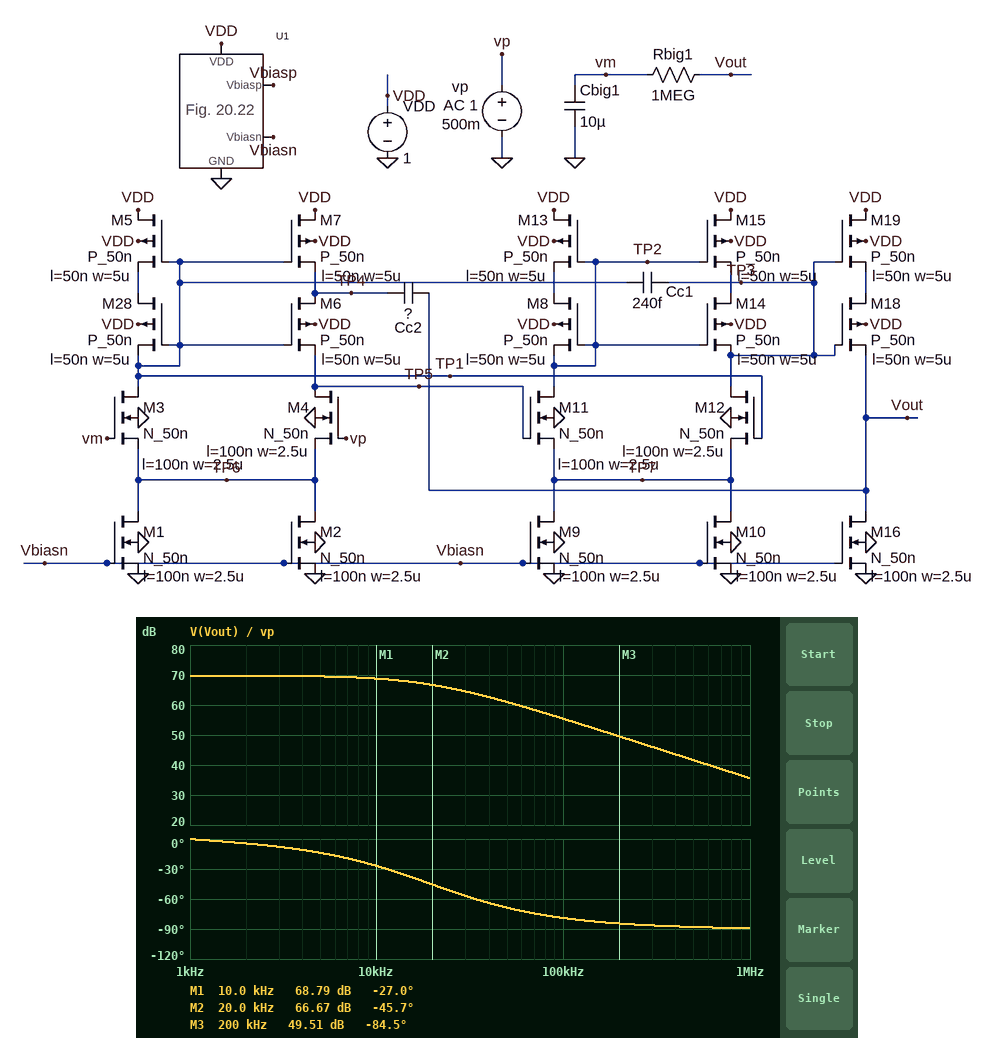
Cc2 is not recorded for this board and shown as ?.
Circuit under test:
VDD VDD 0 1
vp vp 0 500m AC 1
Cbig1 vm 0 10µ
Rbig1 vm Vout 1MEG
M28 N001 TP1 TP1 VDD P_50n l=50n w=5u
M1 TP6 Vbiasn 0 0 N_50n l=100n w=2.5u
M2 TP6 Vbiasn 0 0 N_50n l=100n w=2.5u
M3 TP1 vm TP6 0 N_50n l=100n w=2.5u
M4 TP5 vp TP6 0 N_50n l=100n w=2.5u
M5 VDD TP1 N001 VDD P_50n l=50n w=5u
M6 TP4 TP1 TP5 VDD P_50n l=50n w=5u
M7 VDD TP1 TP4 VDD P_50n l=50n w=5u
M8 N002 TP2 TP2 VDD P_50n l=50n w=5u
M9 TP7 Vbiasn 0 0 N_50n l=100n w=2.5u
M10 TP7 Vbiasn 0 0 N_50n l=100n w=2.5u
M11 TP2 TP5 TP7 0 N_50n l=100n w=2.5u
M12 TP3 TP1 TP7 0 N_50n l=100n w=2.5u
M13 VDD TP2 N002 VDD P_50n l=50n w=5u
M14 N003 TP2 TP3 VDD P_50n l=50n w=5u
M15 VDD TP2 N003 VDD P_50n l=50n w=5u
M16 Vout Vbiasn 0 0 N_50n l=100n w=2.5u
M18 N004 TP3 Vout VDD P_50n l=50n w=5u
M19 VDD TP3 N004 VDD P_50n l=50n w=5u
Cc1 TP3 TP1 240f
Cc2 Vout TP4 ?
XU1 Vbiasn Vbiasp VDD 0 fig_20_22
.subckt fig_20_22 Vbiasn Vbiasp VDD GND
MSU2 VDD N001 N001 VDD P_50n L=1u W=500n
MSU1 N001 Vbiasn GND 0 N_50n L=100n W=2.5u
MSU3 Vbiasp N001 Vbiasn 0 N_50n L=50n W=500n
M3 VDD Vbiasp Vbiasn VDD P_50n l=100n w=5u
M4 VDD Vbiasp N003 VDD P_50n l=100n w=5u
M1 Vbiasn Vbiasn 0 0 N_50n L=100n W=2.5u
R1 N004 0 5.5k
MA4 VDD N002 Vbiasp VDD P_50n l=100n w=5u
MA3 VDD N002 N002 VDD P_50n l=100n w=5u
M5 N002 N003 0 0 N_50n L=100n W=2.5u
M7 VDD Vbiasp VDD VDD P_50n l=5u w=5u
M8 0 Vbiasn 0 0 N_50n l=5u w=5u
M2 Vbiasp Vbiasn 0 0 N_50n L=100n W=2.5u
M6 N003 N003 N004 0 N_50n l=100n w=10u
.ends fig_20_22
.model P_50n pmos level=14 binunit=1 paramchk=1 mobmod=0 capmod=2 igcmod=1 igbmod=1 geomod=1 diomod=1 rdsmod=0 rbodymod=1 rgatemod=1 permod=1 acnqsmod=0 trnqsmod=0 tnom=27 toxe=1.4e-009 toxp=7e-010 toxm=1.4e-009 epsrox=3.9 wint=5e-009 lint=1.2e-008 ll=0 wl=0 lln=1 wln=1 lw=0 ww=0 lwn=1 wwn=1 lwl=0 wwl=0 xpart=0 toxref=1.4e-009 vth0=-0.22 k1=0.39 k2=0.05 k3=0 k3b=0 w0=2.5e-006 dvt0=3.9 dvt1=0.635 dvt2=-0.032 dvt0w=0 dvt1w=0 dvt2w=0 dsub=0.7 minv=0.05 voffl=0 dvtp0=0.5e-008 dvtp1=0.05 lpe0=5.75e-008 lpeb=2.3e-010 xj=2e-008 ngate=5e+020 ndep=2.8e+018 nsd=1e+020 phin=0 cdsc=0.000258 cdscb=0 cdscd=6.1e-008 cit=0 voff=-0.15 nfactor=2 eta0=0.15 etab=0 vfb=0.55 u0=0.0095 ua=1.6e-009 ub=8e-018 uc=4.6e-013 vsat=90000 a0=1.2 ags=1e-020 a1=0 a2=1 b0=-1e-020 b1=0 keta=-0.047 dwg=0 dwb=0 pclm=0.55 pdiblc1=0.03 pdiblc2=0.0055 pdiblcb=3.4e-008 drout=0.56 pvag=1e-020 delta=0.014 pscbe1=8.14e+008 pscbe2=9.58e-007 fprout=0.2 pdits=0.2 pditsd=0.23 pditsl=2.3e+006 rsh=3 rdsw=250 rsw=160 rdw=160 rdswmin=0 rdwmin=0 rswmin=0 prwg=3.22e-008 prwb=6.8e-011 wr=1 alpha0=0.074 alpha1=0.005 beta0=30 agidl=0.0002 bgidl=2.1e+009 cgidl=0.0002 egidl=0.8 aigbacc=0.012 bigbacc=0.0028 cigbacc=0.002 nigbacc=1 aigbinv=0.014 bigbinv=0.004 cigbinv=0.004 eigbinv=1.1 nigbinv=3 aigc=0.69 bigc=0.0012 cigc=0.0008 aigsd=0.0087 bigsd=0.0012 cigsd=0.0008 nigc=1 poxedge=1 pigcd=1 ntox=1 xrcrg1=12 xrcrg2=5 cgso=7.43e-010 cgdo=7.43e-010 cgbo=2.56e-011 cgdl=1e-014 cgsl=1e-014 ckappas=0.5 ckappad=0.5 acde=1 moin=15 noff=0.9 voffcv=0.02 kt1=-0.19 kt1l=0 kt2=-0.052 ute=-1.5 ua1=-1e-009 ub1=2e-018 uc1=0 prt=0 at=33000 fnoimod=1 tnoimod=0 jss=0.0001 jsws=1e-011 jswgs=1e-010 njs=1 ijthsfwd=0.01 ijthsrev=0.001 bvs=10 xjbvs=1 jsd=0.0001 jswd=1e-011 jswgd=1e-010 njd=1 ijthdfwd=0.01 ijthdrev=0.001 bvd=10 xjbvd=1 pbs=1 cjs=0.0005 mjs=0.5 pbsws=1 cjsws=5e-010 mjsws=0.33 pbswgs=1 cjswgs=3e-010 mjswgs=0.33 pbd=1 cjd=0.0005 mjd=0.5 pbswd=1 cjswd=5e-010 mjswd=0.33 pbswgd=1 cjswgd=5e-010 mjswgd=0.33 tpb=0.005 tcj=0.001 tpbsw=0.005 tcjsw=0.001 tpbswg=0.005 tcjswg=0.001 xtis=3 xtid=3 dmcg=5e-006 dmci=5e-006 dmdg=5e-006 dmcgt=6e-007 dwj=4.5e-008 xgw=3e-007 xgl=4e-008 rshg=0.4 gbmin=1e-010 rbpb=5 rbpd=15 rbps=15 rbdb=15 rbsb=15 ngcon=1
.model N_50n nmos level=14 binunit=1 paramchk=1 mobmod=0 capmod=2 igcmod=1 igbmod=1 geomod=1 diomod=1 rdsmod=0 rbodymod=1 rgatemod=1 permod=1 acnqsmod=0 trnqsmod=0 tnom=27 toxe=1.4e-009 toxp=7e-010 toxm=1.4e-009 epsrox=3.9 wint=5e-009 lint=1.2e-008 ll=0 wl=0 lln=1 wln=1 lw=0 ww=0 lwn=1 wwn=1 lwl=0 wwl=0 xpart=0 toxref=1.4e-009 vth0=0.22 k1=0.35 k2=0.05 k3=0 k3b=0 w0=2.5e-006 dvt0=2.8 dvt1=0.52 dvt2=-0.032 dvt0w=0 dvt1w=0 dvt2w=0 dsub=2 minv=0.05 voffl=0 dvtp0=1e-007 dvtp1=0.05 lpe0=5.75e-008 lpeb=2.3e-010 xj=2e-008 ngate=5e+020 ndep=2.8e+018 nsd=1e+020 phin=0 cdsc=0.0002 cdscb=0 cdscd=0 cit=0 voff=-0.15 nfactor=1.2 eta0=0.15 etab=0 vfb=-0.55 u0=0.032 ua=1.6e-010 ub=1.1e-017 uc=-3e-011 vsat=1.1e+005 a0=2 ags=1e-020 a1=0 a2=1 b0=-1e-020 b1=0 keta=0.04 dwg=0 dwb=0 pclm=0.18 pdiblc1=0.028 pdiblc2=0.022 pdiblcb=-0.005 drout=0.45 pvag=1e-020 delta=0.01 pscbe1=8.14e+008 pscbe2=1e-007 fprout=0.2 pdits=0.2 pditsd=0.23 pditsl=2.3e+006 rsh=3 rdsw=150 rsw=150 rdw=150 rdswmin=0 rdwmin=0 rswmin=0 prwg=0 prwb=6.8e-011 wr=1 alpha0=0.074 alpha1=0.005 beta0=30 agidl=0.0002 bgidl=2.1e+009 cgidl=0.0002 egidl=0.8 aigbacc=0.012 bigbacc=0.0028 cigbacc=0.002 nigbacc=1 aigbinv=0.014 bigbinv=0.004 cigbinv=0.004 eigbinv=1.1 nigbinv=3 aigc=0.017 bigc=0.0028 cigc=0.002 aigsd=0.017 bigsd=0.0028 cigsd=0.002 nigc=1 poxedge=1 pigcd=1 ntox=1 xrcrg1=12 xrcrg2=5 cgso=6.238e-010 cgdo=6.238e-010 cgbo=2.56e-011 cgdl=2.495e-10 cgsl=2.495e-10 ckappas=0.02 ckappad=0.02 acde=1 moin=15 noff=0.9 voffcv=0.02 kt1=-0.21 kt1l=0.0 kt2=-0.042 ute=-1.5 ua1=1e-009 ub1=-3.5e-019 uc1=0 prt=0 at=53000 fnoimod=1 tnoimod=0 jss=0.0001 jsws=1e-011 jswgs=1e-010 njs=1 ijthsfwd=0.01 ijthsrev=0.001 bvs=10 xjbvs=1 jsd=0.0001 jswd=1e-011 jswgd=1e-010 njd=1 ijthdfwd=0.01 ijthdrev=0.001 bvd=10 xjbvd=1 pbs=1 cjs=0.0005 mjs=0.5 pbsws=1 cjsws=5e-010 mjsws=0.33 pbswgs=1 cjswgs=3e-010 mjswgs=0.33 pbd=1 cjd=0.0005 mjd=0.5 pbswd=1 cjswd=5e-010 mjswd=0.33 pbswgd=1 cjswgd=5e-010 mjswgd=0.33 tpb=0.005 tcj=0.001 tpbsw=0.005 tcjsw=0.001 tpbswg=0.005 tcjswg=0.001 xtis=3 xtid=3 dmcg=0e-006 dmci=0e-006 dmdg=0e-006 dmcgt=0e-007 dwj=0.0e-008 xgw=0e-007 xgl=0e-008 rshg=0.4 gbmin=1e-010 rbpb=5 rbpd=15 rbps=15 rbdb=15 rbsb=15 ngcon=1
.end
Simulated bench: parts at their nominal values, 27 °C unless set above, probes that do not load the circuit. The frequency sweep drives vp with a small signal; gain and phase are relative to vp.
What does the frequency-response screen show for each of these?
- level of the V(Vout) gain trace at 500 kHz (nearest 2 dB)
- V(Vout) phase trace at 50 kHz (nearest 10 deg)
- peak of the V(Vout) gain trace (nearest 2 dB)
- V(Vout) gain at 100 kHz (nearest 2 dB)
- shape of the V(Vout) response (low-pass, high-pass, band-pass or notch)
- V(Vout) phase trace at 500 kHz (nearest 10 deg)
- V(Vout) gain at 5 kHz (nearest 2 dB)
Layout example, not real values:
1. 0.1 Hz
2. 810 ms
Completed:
1. 42 dB
2. -70 deg
3. 70 dB
4. 56 dB
5. low-pass
6. -90 deg
7. 70 dB
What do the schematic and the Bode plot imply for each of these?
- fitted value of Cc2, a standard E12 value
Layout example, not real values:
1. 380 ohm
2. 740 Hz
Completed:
1. 680 fF
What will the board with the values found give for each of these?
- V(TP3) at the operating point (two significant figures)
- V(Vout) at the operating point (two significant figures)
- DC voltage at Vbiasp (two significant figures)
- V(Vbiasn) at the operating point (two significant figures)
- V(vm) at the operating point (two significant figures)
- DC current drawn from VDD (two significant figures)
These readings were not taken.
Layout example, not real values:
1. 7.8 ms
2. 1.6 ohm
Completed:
1. 670 mV
2. 500 mV
3. 650 mV
4. 350 mV
5. 500 mV
6. 96 µA
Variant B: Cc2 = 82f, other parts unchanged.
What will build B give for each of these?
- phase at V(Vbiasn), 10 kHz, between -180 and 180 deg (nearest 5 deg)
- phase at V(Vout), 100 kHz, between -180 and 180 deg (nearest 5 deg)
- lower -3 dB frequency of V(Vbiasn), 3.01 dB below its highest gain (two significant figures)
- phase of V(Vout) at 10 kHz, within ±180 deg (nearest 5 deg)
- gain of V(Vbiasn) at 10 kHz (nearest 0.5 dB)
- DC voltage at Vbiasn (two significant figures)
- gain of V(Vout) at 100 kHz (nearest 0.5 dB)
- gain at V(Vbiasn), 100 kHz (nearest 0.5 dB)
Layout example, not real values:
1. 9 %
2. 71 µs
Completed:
1. 45 deg
2. -40 deg
3. 120 kHz
4. -5 deg
5. -45.5 dB
6. 350 mV
7. 67.5 dB
8. -29.5 dB
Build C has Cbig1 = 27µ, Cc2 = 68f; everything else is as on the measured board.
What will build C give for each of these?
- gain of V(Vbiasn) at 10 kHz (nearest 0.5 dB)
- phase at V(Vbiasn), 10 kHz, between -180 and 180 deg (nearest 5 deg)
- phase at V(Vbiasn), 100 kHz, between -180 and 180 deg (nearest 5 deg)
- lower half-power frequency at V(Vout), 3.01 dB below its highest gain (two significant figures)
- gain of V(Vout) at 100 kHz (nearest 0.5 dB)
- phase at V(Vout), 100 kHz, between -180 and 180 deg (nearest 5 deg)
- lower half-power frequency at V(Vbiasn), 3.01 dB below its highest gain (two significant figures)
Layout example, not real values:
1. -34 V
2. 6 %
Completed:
1. -45.5 dB
2. 45 deg
3. 50 deg
4. 18 Hz
5. 68.0 dB
6. -35 deg
7. 140 kHz
